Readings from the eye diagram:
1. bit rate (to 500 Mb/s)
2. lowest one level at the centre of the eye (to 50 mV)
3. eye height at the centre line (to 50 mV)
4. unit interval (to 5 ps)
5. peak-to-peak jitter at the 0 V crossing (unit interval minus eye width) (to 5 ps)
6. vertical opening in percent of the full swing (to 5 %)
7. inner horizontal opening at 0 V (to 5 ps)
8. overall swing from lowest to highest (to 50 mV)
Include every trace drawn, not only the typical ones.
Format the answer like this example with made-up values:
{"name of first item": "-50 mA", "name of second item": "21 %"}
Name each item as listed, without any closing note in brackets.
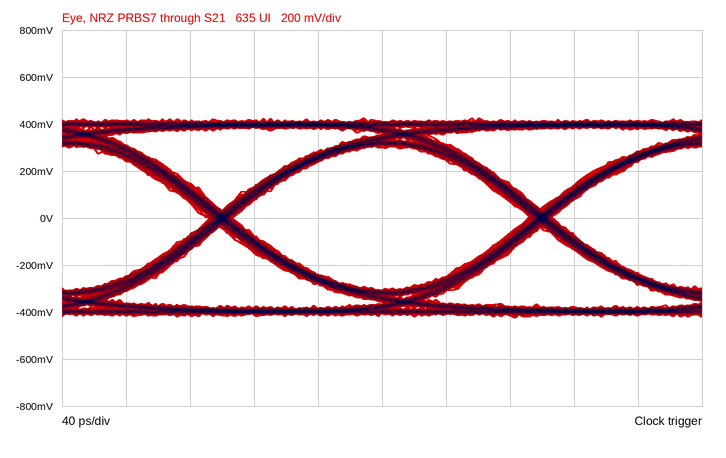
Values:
{"bit rate": "5.0 Gb/s", "lowest one level at the centre of the eye": "300 mV", "eye height at the centre line": "600 mV", "unit interval": "200 ps", "peak-to-peak jitter at the 0 V crossing (unit interval minus eye width)": "15 ps", "vertical opening in percent of the full swing": "70 %", "inner horizontal opening at 0 V": "185 ps", "overall swing from lowest to highest": "850 mV"}
